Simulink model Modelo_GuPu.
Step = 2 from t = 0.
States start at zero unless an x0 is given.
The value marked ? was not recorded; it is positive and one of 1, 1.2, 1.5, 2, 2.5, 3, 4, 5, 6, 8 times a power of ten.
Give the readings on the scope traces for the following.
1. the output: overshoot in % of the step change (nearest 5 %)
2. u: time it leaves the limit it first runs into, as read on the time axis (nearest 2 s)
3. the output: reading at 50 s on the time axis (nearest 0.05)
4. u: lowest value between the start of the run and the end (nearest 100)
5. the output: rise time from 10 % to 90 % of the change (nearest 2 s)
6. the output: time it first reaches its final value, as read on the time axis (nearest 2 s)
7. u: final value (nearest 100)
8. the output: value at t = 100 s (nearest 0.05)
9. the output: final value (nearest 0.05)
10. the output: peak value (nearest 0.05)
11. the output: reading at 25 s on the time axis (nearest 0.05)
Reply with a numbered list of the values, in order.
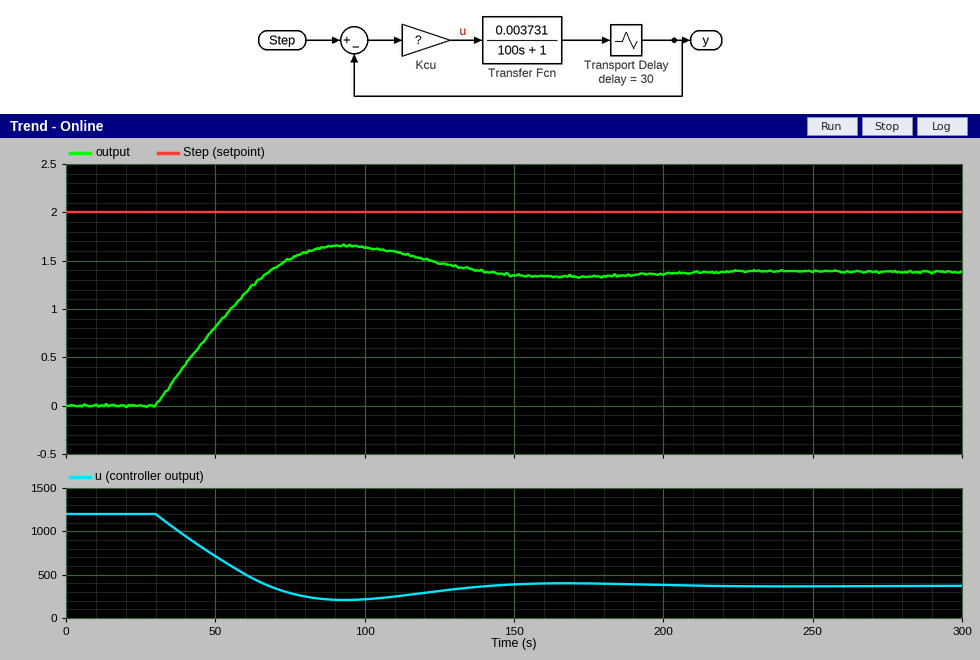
1. 20 %
2. 30 s
3. 0.80
4. 200
5. 30 s
6. 68 s
7. 400
8. 1.65
9. 1.40
10. 1.65
11. 0.00
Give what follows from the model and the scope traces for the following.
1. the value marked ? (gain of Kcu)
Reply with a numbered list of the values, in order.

1. 600
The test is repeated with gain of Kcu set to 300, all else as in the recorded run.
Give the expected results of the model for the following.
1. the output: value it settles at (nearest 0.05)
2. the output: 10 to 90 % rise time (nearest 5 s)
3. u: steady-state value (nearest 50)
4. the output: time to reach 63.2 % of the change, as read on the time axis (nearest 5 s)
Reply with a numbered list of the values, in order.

1. 1.05
2. 60 s
3. 300
4. 65 s
